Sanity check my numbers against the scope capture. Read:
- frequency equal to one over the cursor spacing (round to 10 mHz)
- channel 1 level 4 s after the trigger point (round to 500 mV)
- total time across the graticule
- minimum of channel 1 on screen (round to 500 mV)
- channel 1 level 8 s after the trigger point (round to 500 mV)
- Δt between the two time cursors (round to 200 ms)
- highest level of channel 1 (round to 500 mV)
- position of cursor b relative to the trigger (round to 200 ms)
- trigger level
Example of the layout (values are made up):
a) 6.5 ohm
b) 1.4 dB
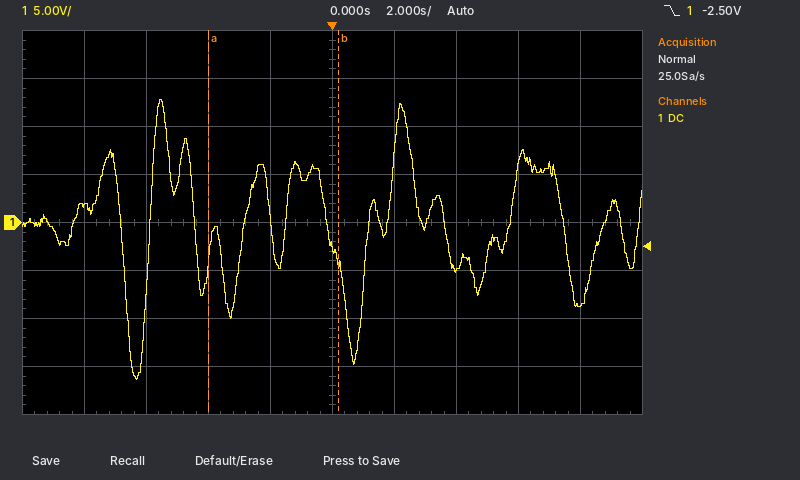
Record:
a) 240 mHz
b) -5.0 V
c) 20 s
d) -16.5 V
e) -8.5 V
f) 4.2 s
g) 13.0 V
h) +200 ms
i) -2.50 V
